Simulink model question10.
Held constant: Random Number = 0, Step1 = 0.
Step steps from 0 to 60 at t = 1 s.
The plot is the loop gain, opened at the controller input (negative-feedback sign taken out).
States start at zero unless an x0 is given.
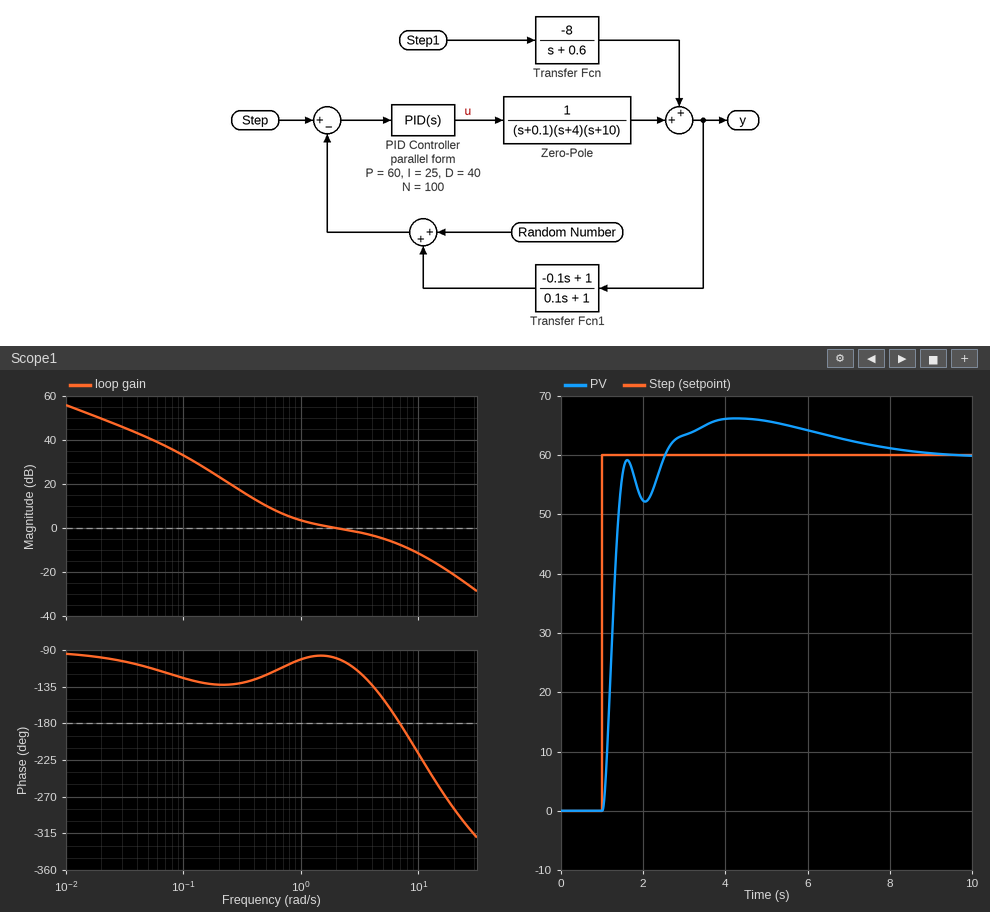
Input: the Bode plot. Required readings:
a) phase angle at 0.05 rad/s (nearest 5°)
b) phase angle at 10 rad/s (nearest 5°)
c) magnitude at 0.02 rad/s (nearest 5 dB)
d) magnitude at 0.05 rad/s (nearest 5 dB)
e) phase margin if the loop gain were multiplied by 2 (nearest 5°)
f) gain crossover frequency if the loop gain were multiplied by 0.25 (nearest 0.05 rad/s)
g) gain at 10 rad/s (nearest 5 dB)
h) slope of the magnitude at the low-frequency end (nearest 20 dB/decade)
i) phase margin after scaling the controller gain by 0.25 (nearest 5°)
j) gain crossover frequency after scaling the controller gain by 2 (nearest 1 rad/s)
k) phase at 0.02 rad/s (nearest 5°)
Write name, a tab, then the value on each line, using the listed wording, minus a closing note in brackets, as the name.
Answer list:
phase angle at 0.05 rad/s	-110°
phase angle at 10 rad/s	-215°
magnitude at 0.02 rad/s	50 dB
magnitude at 0.05 rad/s	40 dB
phase margin if the loop gain were multiplied by 2	15°
gain crossover frequency if the loop gain were multiplied by 0.25	0.45 rad/s
gain at 10 rad/s	-10 dB
slope of the magnitude at the low-frequency end	-20 dB/decade
phase margin after scaling the controller gain by 0.25	55°
gain crossover frequency after scaling the controller gain by 2	6 rad/s
phase at 0.02 rad/s	-100°
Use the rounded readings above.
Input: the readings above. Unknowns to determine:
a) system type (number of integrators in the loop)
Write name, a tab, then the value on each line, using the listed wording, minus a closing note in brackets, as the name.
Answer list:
system type	1
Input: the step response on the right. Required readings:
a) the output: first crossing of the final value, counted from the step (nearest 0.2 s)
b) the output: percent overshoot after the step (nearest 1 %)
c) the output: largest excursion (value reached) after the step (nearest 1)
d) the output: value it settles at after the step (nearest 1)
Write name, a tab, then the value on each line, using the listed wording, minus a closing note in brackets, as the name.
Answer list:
the output: first crossing of the final value, counted from the step	1.6 s
the output: percent overshoot after the step	10 %
the output: largest excursion (value reached) after the step	66
the output: value it settles at after the step	60
